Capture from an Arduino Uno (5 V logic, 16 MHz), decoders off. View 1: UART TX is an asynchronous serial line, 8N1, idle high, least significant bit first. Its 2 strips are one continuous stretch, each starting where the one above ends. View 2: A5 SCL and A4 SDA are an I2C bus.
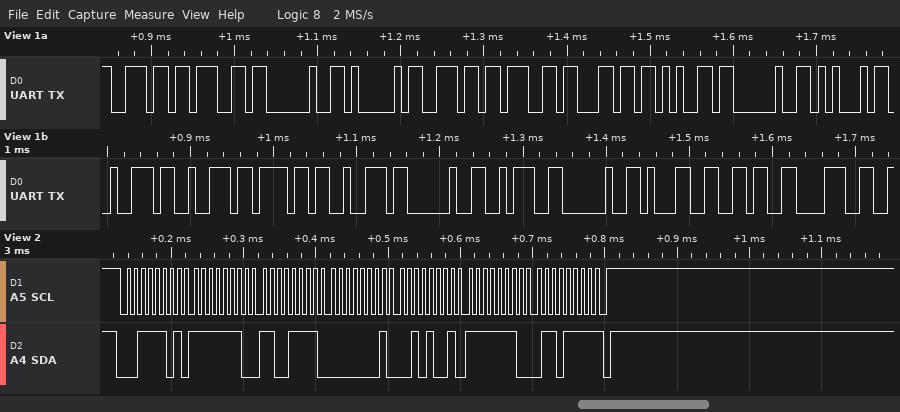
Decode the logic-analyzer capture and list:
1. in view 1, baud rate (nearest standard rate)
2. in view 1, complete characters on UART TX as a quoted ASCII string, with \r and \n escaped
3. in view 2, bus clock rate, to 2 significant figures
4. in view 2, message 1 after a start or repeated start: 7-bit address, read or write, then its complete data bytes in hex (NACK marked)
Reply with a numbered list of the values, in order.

1. 115200 baud
2. "ng Angle Error : 168"
3. 100 kHz
4. 0x1E read: FE CF 01 29 FE 6F NACK
